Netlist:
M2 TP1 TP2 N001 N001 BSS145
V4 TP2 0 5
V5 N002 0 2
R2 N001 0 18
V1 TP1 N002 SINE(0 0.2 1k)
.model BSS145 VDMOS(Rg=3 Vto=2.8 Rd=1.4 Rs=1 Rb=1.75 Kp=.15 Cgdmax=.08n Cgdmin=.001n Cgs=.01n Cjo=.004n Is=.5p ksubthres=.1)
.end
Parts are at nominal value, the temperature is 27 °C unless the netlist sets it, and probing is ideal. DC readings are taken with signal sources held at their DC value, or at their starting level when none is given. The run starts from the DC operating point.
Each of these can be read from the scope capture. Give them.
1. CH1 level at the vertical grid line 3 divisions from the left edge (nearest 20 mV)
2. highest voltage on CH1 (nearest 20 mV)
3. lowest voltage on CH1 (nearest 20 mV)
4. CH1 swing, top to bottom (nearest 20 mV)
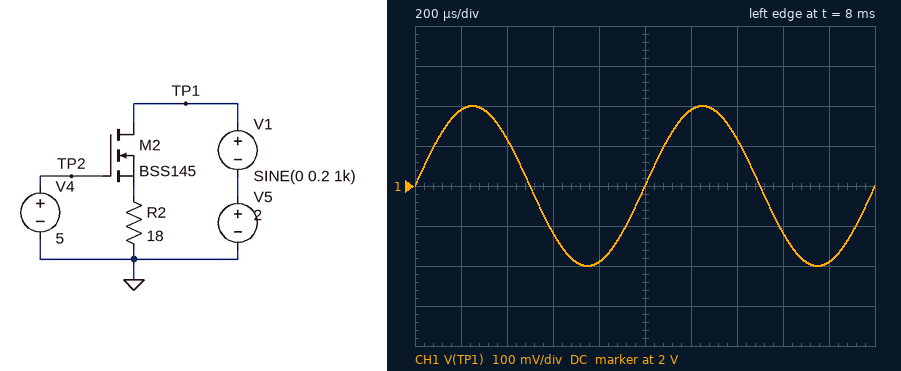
1.88 V
2.20 V
1.80 V
400 mV
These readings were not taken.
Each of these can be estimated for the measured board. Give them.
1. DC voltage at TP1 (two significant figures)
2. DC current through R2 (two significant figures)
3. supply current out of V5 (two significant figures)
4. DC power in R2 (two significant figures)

2.0 V
65 mA
65 mA
75 mW
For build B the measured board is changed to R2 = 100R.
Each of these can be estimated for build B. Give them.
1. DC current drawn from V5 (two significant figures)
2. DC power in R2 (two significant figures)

17 mA
28 mW
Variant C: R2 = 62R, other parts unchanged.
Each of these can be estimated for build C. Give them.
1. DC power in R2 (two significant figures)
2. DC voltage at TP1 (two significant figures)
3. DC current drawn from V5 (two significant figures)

39 mW
2.0 V
25 mA
